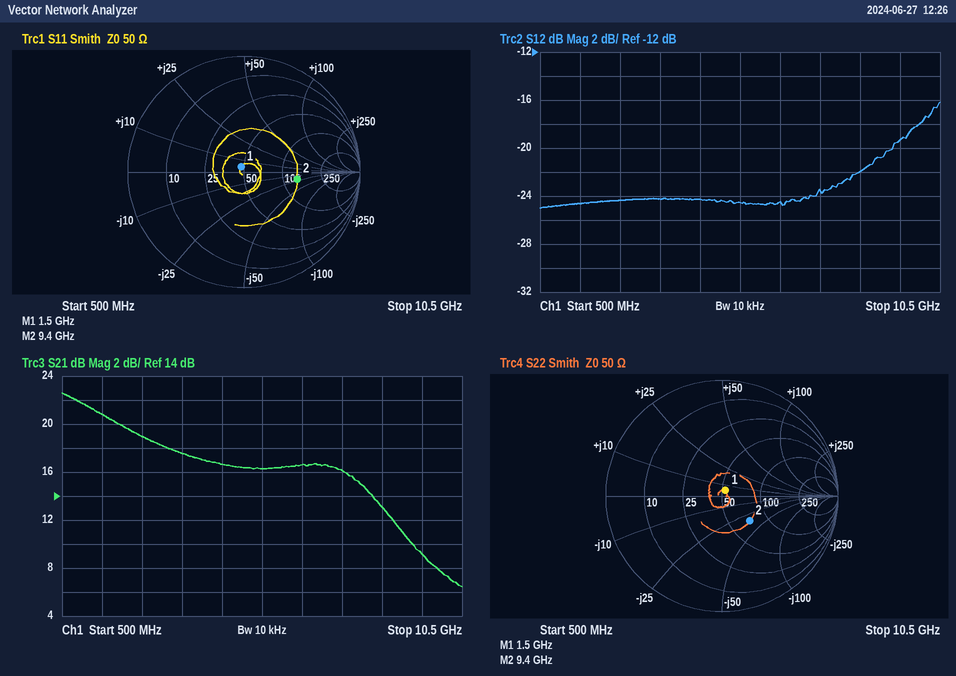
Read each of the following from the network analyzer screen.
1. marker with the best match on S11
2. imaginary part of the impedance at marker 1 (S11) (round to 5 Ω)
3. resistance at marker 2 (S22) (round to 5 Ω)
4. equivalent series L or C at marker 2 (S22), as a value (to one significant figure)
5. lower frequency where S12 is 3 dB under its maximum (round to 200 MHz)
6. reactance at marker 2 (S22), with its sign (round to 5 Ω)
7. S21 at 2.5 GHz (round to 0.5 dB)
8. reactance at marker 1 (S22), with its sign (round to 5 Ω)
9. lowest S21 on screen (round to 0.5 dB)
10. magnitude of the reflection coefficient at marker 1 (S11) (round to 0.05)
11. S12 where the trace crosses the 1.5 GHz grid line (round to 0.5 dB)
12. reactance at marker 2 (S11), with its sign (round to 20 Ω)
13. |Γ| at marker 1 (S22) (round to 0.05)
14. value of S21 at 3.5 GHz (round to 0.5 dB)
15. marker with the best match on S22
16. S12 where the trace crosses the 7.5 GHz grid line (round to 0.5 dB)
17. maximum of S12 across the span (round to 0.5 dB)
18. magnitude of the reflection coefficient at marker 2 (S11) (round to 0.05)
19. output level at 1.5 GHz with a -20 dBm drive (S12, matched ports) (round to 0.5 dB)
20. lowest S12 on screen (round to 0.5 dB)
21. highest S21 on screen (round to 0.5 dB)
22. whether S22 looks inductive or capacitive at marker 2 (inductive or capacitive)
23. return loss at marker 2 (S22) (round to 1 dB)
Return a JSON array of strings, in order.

["marker 1", "+5 Ω", "70 Ω", "500 fF", "9.6 GHz", "-35 Ω", "19.0 dB", "+5 Ω", "6.5 dB", "0.05", "-24.5 dB", "-20 Ω", "0.05", "17.5 dB", "marker 1", "-23.5 dB", "-16.0 dB", "0.45", "-44.5 dBm", "-25.0 dB", "22.5 dB", "capacitive", "10 dB"]
